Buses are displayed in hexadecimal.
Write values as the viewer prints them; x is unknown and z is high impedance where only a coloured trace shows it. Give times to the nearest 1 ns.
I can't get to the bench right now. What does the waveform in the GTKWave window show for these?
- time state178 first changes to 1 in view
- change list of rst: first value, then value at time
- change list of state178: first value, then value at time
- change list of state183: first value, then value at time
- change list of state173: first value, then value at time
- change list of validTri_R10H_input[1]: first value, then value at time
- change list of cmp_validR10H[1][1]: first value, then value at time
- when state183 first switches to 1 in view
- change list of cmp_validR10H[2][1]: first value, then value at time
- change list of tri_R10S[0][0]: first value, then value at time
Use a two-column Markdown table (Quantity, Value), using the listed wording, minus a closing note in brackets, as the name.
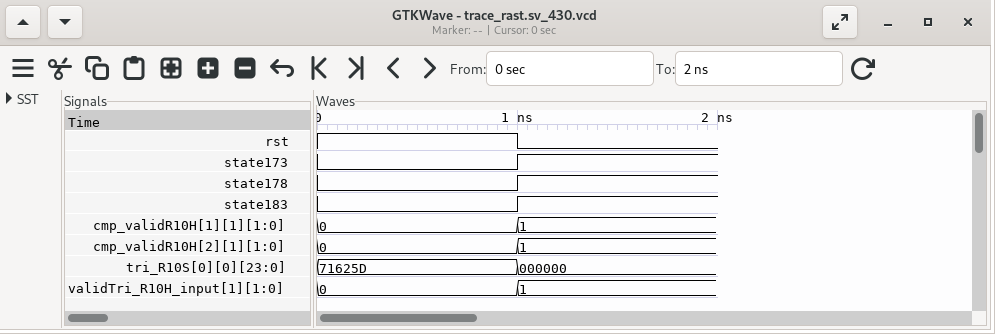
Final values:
| Quantity | Value |
|---|---|
| time state178 first changes to 1 in view | 1 ns |
| change list of rst: first value, then value at time | 1, 0 at 1 ns |
| change list of state178: first value, then value at time | 0, 1 at 1 ns |
| change list of state183: first value, then value at time | 0, 1 at 1 ns |
| change list of state173: first value, then value at time | 0, 1 at 1 ns |
| change list of validTri_R10H_input[1]: first value, then value at time | 0, 1 at 1 ns |
| change list of cmp_validR10H[1][1]: first value, then value at time | 0, 1 at 1 ns |
| when state183 first switches to 1 in view | 1 ns |
| change list of cmp_validR10H[2][1]: first value, then value at time | 0, 1 at 1 ns |
| change list of tri_R10S[0][0]: first value, then value at time | 71625D, 000000 at 1 ns |
